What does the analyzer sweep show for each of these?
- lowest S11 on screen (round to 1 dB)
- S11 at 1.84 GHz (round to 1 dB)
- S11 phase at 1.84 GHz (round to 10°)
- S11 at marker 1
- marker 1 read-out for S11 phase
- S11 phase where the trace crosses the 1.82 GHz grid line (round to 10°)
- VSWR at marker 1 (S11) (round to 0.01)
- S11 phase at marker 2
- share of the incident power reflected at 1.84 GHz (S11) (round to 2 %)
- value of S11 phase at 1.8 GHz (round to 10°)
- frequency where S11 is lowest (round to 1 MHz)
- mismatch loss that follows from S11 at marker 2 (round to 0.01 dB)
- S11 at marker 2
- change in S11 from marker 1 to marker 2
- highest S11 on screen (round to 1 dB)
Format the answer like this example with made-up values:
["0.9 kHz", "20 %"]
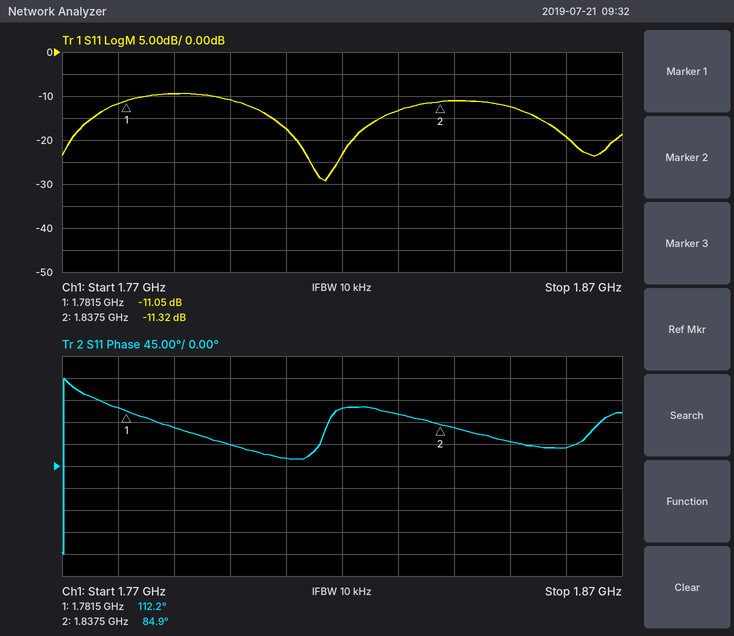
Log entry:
["-29 dB", "-11 dB", "80°", "-11.05 dB", "112.2°", "120°", "1.78", "84.9°", "8 %", "40°", "1.817 GHz", "0.33 dB", "-11.32 dB", "-0.27 dB", "-9 dB"]
